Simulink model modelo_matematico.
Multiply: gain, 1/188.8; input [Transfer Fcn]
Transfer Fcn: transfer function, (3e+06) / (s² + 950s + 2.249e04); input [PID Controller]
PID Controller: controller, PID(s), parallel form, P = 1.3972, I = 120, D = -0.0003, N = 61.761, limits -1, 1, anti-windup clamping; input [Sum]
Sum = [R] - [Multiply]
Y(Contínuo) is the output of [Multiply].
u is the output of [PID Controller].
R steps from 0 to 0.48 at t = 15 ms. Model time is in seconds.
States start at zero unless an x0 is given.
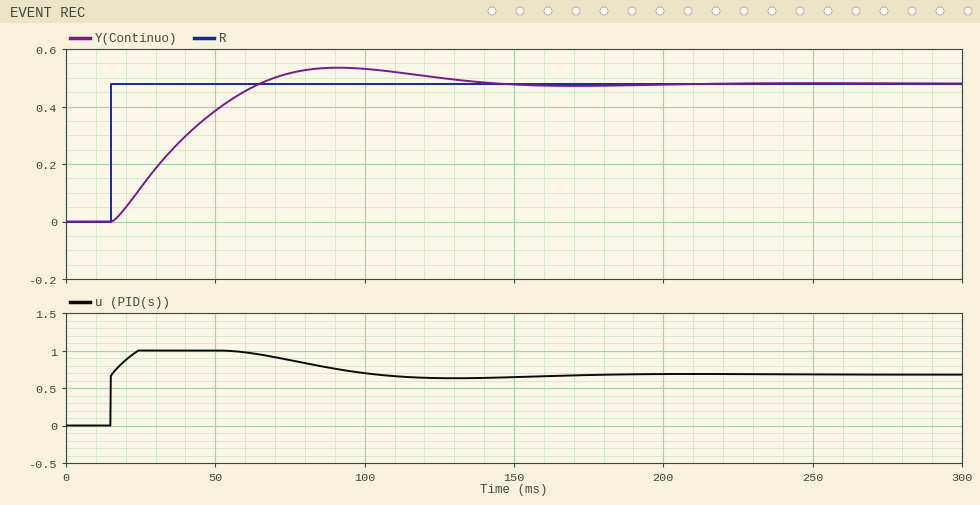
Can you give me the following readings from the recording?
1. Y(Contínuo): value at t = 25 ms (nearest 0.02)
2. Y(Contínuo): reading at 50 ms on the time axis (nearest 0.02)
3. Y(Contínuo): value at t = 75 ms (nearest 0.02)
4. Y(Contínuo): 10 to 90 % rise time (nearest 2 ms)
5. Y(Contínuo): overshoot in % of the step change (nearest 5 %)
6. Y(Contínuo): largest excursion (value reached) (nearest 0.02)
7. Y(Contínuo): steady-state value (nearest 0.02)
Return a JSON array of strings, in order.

["0.12", "0.38", "0.52", "36 ms", "10 %", "0.54", "0.48"]
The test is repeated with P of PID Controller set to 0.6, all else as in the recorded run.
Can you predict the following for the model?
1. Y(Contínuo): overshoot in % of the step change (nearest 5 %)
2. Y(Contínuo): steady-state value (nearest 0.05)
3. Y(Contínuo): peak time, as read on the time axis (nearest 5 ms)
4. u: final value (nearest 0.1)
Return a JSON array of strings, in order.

["15 %", "0.50", "95 ms", "0.7"]
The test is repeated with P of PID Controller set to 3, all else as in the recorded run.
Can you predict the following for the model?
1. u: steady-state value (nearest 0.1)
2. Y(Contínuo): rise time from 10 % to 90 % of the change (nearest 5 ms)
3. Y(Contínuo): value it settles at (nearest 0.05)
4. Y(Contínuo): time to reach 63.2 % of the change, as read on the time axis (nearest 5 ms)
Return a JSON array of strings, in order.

["0.7", "40 ms", "0.50", "40 ms"]
